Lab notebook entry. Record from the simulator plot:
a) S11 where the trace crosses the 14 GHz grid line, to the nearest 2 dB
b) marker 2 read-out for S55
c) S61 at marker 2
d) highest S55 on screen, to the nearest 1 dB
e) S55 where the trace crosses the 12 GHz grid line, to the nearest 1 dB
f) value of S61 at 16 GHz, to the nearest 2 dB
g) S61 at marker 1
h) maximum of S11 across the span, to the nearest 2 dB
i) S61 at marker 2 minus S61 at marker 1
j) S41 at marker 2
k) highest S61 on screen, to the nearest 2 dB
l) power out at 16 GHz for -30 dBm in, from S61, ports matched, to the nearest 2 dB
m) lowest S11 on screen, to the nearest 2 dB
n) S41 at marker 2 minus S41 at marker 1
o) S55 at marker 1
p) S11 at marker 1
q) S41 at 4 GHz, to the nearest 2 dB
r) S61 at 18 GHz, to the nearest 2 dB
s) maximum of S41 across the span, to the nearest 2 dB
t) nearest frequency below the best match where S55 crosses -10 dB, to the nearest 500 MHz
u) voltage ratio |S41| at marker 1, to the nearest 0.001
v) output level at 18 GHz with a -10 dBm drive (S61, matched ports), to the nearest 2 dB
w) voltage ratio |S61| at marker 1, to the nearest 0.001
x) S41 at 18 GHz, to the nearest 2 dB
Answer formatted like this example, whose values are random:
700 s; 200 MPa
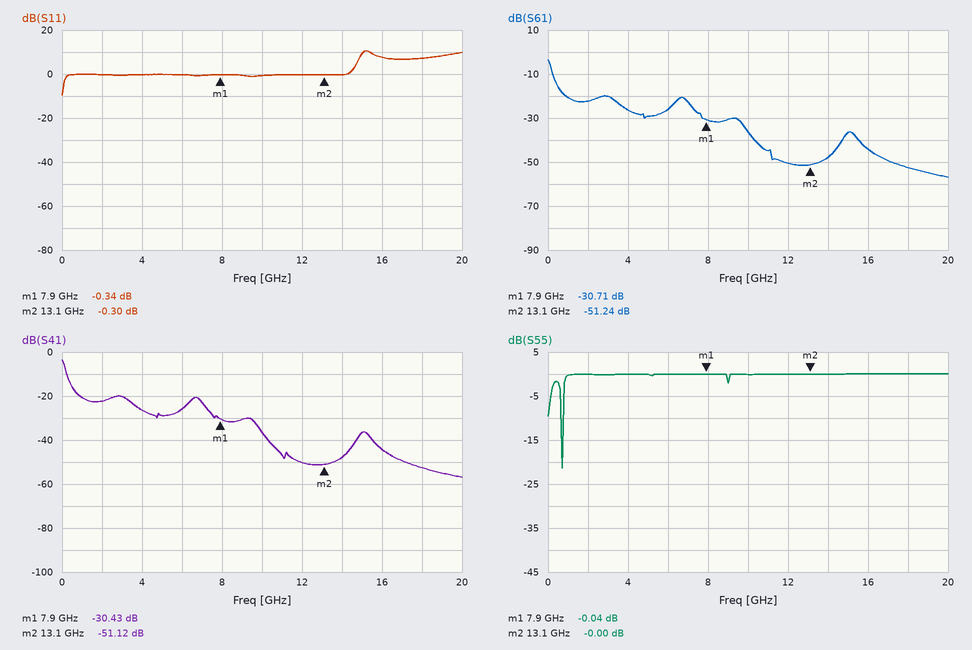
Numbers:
0 dB; -0.00 dB; -51.24 dB; 0 dB; 0 dB; -44 dB; -30.71 dB; 10 dB; -20.53 dB; -51.12 dB; -4 dB; -74 dBm; -10 dB; -20.69 dB; -0.04 dB; -0.34 dB; -26 dB; -52 dB; -4 dB; 500 MHz; 0.030; -62 dBm; 0.029; -52 dB
